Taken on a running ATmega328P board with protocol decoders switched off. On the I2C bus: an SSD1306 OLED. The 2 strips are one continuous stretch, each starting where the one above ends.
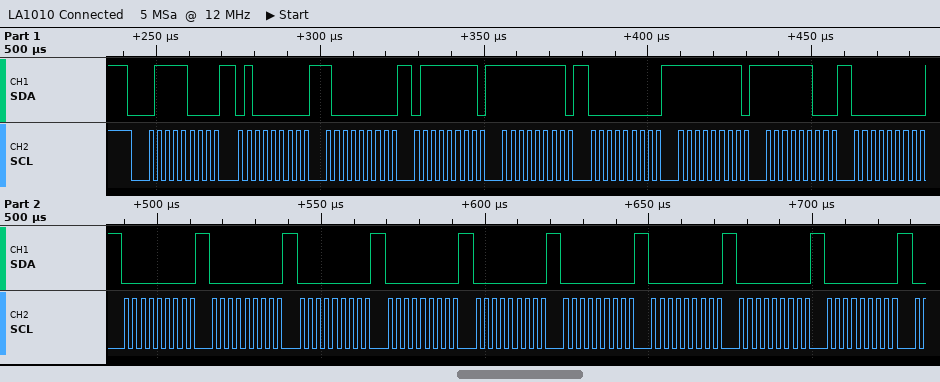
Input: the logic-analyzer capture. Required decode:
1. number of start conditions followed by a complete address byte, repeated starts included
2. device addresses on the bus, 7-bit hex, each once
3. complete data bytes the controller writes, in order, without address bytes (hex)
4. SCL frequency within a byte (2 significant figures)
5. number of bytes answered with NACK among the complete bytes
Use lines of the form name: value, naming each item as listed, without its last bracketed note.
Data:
number of start conditions followed by a complete address byte, repeated starts included: 1
device addresses on the bus, 7-bit hex, each once: 0x3C
complete data bytes the controller writes, in order, without address bytes: 40 80 7F FF 00 FF FC 00 00 00 00 00 00 00 00 00 00
SCL frequency within a byte: 400 kHz
number of bytes answered with NACK among the complete bytes: 0
